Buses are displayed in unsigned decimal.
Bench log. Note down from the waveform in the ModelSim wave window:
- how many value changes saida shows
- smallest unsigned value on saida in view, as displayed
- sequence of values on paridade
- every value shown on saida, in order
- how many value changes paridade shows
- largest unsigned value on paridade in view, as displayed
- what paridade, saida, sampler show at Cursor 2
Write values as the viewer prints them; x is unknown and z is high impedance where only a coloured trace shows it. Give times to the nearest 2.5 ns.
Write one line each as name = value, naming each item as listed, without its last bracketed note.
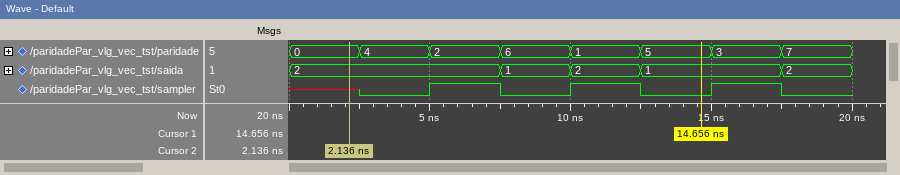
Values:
how many value changes saida shows = 4
smallest unsigned value on saida in view, as displayed = 1
sequence of values on paridade = 0, 4, 2, 6, 1, 5, 3, 7
every value shown on saida, in order = 2, 1, 2, 1, 2
how many value changes paridade shows = 7
largest unsigned value on paridade in view, as displayed = 7
what paridade, saida, sampler show at Cursor 2 = paridade=0, saida=2, sampler=x
